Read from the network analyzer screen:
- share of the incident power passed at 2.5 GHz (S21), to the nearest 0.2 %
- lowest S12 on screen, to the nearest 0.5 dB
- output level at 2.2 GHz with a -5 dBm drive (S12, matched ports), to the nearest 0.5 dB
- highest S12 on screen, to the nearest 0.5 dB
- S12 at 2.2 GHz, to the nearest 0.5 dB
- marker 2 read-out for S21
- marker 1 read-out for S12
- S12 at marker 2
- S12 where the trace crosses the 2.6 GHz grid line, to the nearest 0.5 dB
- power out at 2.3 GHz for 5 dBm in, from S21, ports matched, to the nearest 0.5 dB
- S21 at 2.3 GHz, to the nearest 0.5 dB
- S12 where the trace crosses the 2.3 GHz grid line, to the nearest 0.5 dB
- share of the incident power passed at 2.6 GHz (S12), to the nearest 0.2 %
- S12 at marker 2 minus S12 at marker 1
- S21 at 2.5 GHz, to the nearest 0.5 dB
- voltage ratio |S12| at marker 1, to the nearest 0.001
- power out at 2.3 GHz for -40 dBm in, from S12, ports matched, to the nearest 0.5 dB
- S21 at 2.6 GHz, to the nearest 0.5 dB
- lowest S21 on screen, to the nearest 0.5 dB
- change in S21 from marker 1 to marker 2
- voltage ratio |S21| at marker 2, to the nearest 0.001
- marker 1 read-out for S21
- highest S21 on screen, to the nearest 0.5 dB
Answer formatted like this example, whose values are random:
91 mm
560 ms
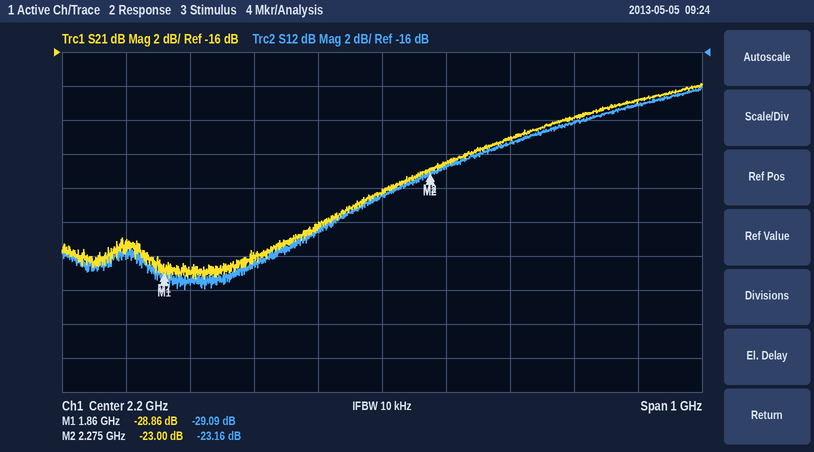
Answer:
1.0 %
-30.0 dB
-29.5 dBm
-18.0 dB
-24.5 dB
-23.00 dB
-29.09 dB
-23.16 dB
-19.0 dB
-17.5 dBm
-22.5 dB
-23.0 dB
1.2 %
5.93 dB
-20.0 dB
0.035
-63.0 dBm
-19.0 dB
-29.5 dB
5.86 dB
0.071
-28.86 dB
-18.0 dB
